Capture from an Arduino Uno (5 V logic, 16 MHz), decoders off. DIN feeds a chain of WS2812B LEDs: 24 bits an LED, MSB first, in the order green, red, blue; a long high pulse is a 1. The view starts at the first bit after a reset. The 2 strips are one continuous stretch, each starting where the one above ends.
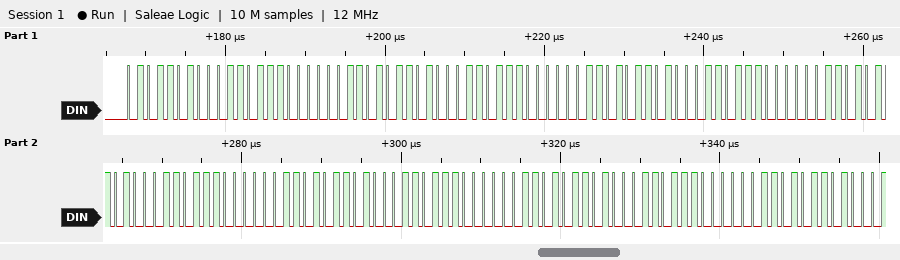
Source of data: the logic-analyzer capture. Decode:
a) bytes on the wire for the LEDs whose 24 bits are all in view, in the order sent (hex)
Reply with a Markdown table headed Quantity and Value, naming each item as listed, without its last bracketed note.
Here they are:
| Quantity | Value |
|---|---|
| bytes on the wire for the LEDs whose 24 bits are all in view, in the order sent | 5A 37 03 5A 37 03 5A 37 03 5A 37 03 5A 37 03 5A 37 03 |
